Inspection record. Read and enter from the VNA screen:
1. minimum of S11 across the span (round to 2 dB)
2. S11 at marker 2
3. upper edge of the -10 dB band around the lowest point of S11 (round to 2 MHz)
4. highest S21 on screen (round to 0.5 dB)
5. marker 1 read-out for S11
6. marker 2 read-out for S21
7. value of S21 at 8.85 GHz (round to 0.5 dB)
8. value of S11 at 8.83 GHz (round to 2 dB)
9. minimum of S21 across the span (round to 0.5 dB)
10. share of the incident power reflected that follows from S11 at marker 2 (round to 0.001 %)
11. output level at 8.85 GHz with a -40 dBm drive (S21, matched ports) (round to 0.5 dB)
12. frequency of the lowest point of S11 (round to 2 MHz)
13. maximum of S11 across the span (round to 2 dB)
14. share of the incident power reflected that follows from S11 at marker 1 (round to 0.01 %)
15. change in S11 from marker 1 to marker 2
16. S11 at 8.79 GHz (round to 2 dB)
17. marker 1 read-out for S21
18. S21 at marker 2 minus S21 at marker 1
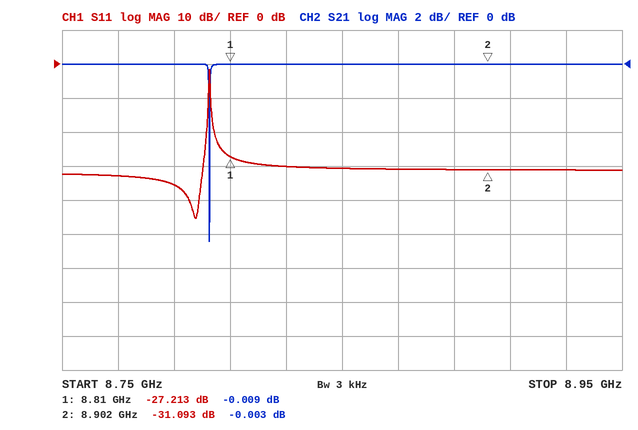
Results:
-46 dB
-31.093 dB
8.802 GHz
0.0 dB
-27.213 dB
-0.003 dB
0.0 dB
-30 dB
-10.5 dB
0.078 %
-40.0 dBm
8.798 GHz
-2 dB
0.19 %
-3.880 dB
-36 dB
-0.009 dB
0.006 dB
